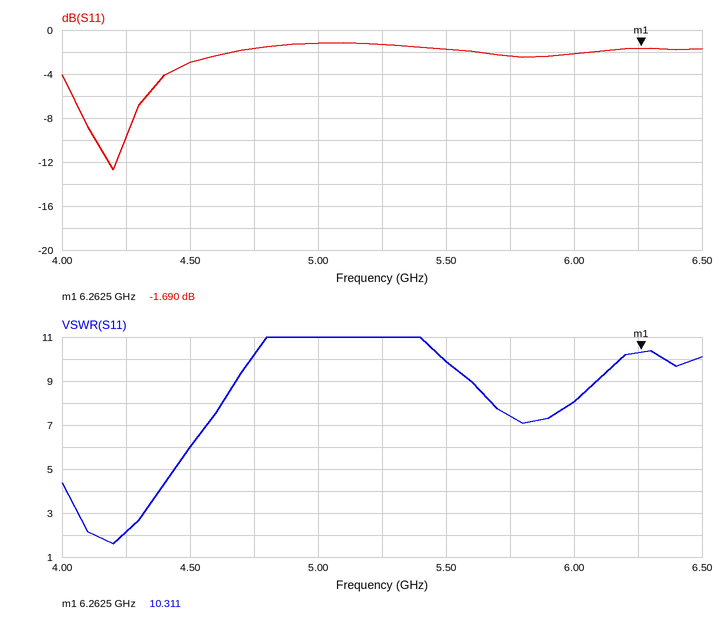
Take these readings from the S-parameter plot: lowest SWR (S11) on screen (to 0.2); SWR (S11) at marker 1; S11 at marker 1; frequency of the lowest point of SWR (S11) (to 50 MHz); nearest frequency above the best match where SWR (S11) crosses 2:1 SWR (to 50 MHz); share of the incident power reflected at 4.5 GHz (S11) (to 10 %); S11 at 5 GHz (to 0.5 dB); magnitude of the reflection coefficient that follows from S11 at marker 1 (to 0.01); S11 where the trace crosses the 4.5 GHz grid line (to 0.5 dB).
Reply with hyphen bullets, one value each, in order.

- 1.6
- 10.311
- -1.690 dB
- 4.20 GHz
- 4.25 GHz
- 50 %
- -1.0 dB
- 0.82
- -3.0 dB
